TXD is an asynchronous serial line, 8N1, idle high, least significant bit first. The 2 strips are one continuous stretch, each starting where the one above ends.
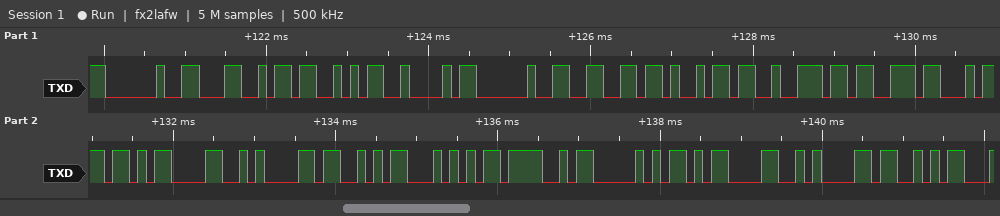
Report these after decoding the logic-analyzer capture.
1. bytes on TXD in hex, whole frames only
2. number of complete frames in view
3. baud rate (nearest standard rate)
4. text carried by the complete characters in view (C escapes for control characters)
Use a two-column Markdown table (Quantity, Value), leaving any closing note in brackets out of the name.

| Quantity | Value |
|---|---|
| bytes on TXD in hex, whole frames only | 20 4C 53 42 20 66 69 72 73 74 0D 0A 53 54 4F 50 0D 0A 53 |
| number of complete frames in view | 19 |
| baud rate | 9600 baud |
| text carried by the complete characters in view | " LSB first\r\nSTOP\r\nS" |
